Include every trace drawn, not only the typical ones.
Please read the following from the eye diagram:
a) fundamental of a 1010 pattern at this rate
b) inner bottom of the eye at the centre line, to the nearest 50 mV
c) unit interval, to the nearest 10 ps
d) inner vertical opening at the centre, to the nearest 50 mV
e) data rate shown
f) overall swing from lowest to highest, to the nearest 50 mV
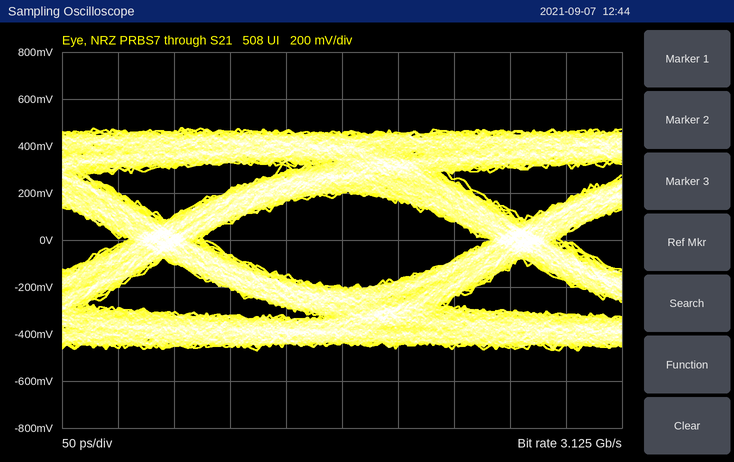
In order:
1.5625 GHz
-200 mV
320 ps
400 mV
3.125 Gb/s
950 mV
